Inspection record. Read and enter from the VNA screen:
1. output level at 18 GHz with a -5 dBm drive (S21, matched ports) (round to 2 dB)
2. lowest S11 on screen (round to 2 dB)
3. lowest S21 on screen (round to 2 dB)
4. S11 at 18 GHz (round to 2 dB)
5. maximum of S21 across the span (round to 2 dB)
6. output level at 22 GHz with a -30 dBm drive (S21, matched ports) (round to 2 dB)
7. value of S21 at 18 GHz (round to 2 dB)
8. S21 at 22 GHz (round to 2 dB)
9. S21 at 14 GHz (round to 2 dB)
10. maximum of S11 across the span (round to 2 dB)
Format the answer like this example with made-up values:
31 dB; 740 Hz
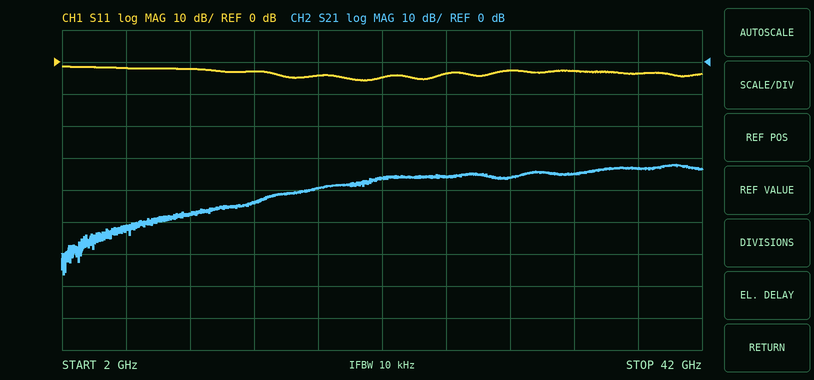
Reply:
-44 dBm; -6 dB; -66 dB; -4 dB; -32 dB; -66 dBm; -40 dB; -36 dB; -44 dB; -2 dB
